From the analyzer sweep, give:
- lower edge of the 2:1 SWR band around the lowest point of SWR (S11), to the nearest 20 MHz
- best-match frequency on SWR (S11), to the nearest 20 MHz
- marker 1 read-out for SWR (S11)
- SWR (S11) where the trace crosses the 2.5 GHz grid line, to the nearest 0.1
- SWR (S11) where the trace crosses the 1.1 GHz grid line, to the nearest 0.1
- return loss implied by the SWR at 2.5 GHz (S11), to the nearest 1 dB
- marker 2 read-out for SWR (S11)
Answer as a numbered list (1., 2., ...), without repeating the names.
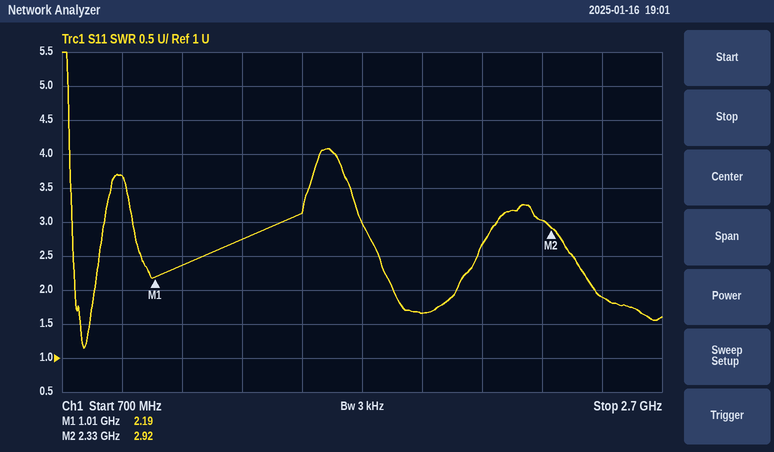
1. 740 MHz
2. 780 MHz
3. 2.19
4. 1.9
5. 2.4
6. 10 dB
7. 2.92
